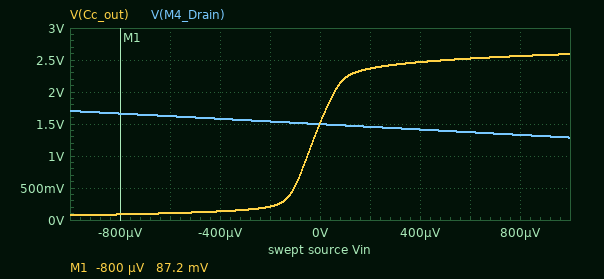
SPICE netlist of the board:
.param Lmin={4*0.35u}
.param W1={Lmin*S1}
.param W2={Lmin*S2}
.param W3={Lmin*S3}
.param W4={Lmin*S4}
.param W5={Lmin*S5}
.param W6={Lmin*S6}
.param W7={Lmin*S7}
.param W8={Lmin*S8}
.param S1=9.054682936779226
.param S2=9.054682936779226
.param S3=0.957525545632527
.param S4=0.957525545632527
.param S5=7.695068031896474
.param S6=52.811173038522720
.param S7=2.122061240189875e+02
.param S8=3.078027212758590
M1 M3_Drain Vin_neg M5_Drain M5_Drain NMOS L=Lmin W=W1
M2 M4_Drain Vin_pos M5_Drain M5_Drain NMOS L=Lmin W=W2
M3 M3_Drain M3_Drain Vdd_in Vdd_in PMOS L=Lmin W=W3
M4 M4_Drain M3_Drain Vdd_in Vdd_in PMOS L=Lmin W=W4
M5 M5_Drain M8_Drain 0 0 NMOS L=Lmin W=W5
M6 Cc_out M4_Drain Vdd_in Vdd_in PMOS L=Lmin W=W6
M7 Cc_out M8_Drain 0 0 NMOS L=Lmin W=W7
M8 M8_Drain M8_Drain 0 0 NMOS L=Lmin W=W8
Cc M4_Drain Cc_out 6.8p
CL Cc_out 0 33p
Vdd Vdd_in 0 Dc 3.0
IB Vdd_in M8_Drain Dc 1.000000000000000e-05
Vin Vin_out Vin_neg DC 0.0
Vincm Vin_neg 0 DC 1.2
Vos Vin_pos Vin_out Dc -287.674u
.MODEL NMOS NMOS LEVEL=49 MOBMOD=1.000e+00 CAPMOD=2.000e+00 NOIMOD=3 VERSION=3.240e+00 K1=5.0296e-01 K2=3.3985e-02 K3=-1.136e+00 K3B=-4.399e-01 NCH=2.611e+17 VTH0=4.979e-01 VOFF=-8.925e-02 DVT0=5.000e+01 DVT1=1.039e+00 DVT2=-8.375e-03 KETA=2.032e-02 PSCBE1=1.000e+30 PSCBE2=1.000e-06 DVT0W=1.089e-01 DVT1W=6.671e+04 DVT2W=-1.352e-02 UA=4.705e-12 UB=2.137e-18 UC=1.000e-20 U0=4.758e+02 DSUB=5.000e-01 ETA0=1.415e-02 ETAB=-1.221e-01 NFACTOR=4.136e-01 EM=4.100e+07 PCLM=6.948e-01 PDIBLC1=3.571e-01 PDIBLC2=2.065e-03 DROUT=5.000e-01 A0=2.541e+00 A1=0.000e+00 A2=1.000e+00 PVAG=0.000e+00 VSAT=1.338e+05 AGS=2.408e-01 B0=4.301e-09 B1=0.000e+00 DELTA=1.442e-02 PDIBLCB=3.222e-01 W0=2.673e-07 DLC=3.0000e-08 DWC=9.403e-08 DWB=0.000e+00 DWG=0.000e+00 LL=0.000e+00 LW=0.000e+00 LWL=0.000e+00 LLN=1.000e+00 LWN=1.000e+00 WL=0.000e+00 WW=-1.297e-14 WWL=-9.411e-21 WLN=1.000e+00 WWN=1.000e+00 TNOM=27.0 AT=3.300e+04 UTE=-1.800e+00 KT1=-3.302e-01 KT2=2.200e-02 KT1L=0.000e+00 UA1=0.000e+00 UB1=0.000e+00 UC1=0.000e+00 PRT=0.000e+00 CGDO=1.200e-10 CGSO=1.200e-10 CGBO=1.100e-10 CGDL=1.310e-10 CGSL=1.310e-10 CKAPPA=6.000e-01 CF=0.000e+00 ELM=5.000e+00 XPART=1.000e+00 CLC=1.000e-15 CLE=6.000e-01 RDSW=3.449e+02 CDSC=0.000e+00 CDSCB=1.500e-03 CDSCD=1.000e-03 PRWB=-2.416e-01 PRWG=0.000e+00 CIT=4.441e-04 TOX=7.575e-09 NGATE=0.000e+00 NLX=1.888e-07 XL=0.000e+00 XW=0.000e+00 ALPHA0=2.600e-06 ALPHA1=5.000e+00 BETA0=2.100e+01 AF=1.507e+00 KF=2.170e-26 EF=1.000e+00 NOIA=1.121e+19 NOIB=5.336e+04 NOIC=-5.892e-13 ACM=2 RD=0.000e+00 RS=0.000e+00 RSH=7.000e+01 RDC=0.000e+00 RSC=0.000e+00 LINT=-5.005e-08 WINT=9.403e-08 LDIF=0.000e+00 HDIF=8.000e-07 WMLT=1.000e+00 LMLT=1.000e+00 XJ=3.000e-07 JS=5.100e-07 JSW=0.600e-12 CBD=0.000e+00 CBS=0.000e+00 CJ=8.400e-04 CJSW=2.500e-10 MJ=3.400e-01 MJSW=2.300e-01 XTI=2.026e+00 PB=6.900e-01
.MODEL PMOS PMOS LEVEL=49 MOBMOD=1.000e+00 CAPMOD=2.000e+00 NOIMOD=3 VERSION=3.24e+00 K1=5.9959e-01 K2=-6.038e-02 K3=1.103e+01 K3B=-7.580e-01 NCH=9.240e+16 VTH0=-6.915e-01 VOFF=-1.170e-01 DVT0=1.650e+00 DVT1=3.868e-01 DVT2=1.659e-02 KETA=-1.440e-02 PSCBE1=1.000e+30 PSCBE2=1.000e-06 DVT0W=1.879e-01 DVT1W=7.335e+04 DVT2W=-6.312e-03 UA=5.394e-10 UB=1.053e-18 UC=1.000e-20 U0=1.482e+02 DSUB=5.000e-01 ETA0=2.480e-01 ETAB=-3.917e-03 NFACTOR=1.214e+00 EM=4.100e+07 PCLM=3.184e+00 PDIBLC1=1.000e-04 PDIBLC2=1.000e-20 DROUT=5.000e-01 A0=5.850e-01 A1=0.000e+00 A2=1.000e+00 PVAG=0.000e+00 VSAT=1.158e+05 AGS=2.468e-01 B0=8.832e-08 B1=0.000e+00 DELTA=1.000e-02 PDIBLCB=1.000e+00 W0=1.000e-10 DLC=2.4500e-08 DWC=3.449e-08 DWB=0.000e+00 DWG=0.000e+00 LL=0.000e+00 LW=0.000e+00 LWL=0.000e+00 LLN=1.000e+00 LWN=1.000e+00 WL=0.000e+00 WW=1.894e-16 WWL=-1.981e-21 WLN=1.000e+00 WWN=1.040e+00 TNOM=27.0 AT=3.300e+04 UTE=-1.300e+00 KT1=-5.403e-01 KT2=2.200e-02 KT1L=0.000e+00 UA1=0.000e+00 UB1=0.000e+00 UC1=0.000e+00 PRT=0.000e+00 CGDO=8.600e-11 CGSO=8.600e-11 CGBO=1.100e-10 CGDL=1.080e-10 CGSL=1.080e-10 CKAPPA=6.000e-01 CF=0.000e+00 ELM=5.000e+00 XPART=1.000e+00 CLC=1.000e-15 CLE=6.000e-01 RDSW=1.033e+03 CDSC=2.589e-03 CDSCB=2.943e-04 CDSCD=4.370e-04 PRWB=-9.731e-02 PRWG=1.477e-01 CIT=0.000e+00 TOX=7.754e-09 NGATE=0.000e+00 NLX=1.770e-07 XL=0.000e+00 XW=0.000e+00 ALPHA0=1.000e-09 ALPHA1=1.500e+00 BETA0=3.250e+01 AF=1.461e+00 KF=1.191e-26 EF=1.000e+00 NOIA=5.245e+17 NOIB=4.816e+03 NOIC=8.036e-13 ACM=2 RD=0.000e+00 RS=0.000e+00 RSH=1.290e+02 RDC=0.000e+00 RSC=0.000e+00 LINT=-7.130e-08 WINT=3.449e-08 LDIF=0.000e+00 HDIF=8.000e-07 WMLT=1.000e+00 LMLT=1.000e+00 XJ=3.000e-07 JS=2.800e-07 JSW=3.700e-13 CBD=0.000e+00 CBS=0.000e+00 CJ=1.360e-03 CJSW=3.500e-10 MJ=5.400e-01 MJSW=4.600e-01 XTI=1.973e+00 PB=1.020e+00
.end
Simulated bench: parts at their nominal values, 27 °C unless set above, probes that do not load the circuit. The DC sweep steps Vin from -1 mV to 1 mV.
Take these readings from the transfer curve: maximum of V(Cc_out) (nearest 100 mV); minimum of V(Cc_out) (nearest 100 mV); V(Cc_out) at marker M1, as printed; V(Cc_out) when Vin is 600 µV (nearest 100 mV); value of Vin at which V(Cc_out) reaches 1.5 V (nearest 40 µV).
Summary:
2.6 V
100 mV
87.2 mV
2.5 V
0 V
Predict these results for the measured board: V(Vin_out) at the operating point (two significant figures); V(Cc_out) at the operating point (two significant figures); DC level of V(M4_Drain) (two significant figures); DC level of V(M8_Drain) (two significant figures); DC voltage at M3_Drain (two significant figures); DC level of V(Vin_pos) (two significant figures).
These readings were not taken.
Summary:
1.2 V
1.5 V
1.5 V
740 mV
1.4 V
1.2 V
